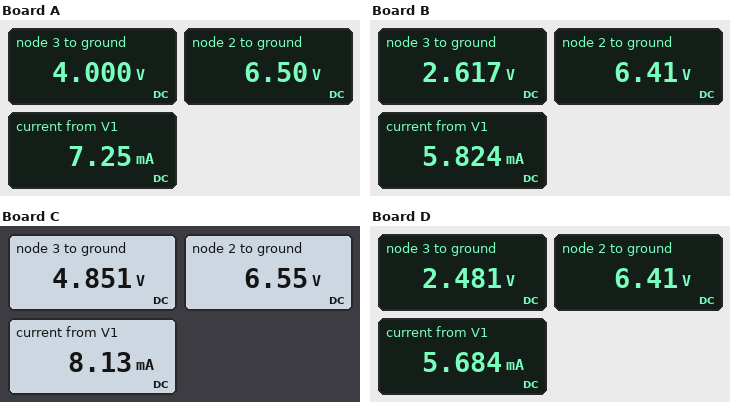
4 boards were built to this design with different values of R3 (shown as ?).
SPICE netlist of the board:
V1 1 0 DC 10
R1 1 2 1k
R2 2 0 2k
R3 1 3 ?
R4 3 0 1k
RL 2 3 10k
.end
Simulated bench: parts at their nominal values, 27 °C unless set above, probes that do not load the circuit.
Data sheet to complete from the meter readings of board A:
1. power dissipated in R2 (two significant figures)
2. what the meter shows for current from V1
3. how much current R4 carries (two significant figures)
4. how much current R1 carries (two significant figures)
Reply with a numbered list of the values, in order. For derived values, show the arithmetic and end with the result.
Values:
1. (6.5 V)^2 / 2 kΩ = 21 mW
2. 7.25 mA
3. (4 V) / 1 kΩ = 4.0 mA
4. (10 V - 6.5 V) / 1 kΩ = 3.5 mA
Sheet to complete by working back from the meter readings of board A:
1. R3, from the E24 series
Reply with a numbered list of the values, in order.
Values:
1. 1.6 kΩ
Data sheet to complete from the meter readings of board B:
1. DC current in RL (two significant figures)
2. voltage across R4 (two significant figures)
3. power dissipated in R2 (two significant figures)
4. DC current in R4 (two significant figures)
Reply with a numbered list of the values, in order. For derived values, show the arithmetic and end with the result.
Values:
1. (6.41 V - 2.617 V) / 10 kΩ = 380 µA
2. 2.617 V = 2.6 V
3. (6.41 V)^2 / 2 kΩ = 21 mW
4. (2.617 V) / 1 kΩ = 2.6 mA
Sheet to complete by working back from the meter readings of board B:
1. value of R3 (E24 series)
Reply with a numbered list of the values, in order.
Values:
1. 3.3 kΩ
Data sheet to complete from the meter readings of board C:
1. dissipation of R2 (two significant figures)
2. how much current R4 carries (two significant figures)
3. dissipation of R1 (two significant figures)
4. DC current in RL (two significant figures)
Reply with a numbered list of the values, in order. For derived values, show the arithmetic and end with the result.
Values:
1. (6.55 V)^2 / 2 kΩ = 21 mW
2. (4.851 V) / 1 kΩ = 4.9 mA
3. (10 V - 6.55 V)^2 / 1 kΩ = 12 mW
4. (6.55 V - 4.851 V) / 10 kΩ = 170 µA
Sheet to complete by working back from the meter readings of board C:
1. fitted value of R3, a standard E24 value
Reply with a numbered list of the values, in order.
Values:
1. 1.1 kΩ
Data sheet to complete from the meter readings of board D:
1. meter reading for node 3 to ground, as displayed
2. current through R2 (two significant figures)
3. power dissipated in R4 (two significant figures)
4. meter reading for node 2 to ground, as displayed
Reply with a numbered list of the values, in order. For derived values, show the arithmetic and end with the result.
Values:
1. 2.481 V
2. (6.41 V) / 2 kΩ = 3.2 mA
3. (2.481 V)^2 / 1 kΩ = 6.2 mW
4. 6.41 V
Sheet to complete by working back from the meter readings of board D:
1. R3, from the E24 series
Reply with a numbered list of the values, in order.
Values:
1. 3.6 kΩ
